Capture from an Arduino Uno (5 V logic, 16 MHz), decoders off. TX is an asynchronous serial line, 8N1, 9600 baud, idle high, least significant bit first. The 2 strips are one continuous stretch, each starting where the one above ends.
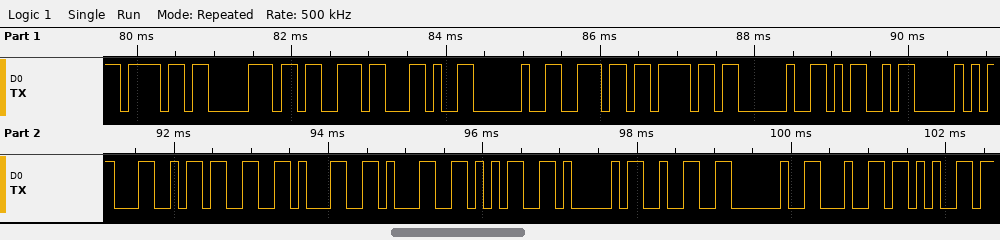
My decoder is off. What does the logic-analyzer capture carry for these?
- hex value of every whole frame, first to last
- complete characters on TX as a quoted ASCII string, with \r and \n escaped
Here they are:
6F 70 73 2C 20 6E 6F 20 4D 50 4C 33 31 31 35 41 32 20 64 65
"ops, no MPL3115A2 de"
